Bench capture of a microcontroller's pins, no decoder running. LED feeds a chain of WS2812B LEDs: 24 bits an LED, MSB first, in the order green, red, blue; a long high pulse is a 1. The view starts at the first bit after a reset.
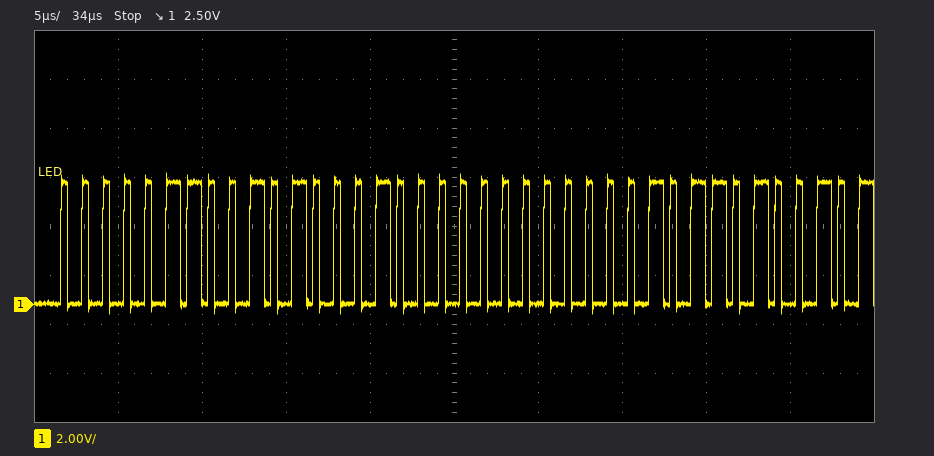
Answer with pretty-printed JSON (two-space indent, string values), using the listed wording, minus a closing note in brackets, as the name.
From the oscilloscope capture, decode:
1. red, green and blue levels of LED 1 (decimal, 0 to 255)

{
  "red, green and blue levels of LED 1": "81, 6, 0"
}
